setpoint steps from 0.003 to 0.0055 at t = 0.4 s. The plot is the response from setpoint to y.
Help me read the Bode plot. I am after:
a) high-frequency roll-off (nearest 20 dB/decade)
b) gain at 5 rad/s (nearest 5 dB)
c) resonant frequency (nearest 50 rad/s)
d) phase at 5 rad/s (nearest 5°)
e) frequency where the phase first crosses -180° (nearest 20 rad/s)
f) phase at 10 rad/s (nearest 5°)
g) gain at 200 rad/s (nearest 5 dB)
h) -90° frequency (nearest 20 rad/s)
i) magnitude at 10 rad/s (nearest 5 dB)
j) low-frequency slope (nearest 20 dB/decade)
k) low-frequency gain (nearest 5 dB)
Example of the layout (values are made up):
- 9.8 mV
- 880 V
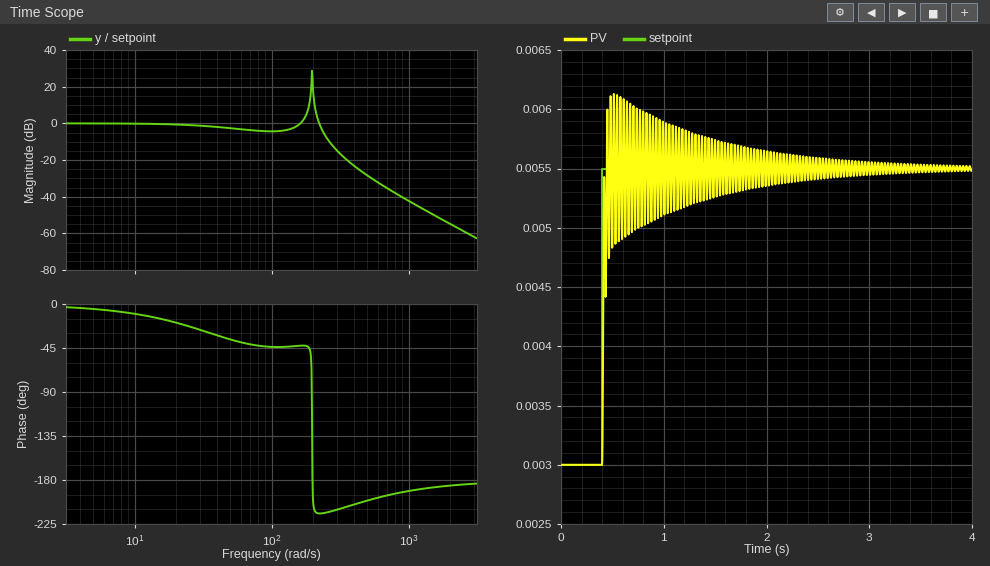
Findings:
- -40 dB/decade
- 0 dB
- 200 rad/s
- -5°
- 200 rad/s
- -10°
- 20 dB
- 200 rad/s
- 0 dB
- 0 dB/decade
- 0 dB
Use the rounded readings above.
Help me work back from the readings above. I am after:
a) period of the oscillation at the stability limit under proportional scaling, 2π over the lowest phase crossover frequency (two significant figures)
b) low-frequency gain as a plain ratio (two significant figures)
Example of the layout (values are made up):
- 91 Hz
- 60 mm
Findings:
- 0.031 s
- 1.0
